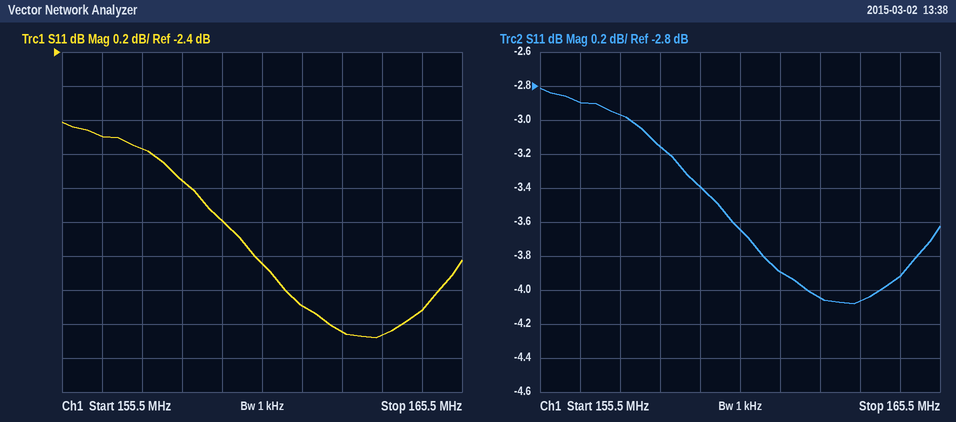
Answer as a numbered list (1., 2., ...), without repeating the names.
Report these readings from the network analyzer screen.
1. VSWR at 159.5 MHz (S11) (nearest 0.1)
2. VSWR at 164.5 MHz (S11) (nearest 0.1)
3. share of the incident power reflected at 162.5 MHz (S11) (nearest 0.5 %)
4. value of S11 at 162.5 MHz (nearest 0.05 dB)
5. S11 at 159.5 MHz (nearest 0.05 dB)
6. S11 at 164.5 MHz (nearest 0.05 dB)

1. 5.2
2. 4.5
3. 39.5 %
4. -4.05 dB
5. -3.40 dB
6. -3.90 dB
